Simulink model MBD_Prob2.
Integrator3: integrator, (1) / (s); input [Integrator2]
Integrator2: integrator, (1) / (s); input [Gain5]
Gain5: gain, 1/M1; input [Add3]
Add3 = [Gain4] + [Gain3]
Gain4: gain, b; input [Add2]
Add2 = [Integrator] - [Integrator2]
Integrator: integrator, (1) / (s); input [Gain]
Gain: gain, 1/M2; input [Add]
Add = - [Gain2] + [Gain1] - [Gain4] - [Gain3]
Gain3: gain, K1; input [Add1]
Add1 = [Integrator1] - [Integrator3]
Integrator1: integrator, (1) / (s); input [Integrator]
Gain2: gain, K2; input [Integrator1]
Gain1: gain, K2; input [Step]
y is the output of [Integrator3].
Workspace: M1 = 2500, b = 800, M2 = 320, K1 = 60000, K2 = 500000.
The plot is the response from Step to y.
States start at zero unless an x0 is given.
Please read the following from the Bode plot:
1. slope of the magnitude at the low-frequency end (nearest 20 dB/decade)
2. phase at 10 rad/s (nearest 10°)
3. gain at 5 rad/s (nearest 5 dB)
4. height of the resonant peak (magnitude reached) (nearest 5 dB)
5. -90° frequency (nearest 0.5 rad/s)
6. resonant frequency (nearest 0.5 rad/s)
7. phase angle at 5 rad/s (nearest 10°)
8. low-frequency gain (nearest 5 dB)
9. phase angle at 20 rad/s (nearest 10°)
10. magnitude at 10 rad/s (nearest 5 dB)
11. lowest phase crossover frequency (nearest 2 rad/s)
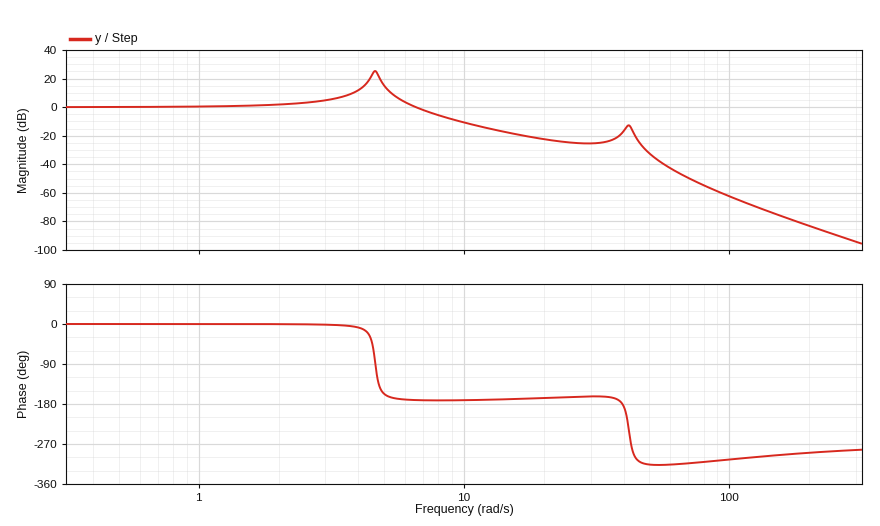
0 dB/decade
-170°
15 dB
25 dB
4.5 rad/s
4.5 rad/s
-160°
0 dB
-170°
-10 dB
40 rad/s
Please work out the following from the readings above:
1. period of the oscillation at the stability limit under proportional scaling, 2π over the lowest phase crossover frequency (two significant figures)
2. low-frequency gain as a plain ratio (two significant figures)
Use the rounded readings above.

0.16 s
1.0
